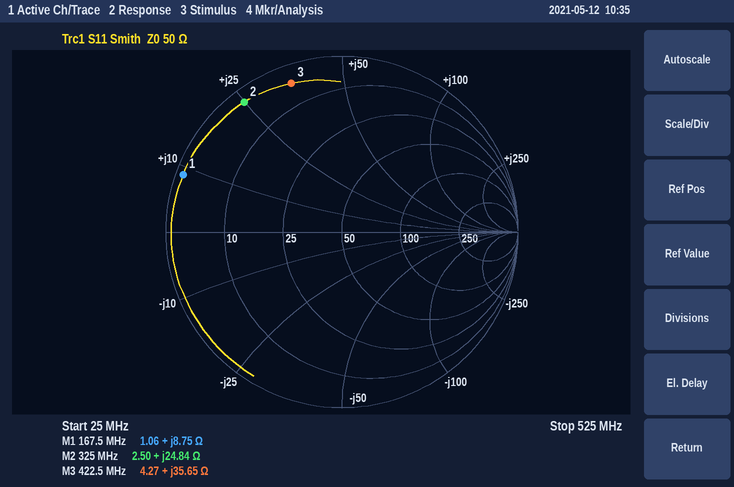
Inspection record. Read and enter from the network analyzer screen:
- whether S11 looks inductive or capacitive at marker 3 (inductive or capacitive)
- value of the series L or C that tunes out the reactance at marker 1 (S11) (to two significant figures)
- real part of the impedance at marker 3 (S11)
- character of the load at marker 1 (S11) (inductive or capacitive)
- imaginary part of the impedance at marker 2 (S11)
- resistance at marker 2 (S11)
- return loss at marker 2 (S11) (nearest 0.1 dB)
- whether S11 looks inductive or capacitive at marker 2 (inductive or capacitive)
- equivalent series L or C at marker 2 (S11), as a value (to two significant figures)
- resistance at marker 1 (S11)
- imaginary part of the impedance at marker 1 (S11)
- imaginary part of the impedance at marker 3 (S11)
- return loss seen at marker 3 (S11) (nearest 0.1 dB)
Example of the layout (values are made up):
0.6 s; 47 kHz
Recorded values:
inductive; 110 pF; 4.27 Ω; inductive; +24.84 Ω; 2.50 Ω; 0.7 dB; inductive; 12 nH; 1.06 Ω; +8.75 Ω; +35.65 Ω; 1.0 dB
